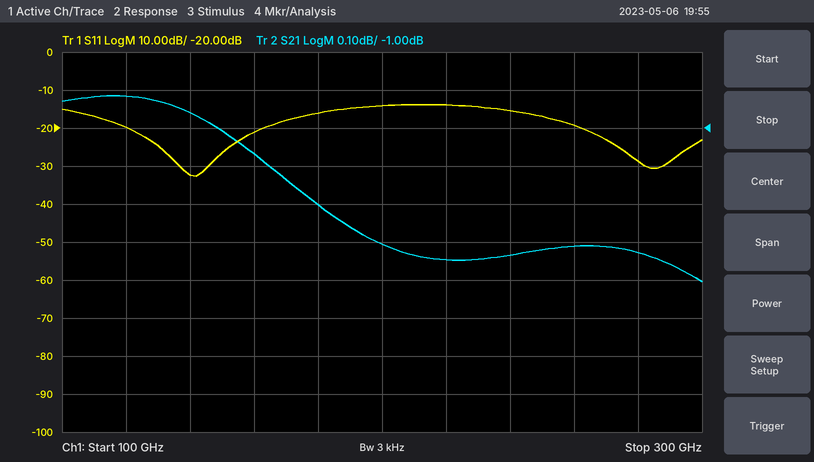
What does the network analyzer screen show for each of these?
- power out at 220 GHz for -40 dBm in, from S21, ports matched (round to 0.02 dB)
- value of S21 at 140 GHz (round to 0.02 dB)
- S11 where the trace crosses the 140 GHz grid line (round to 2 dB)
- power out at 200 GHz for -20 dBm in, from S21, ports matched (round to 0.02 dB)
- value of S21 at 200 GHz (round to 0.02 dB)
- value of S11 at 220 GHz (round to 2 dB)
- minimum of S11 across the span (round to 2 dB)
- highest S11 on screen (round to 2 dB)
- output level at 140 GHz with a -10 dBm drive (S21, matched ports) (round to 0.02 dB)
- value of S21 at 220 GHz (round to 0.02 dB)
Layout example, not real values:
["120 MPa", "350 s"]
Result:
["-41.34 dBm", "-0.96 dB", "-32 dB", "-21.30 dBm", "-1.30 dB", "-14 dB", "-32 dB", "-14 dB", "-10.96 dBm", "-1.34 dB"]
